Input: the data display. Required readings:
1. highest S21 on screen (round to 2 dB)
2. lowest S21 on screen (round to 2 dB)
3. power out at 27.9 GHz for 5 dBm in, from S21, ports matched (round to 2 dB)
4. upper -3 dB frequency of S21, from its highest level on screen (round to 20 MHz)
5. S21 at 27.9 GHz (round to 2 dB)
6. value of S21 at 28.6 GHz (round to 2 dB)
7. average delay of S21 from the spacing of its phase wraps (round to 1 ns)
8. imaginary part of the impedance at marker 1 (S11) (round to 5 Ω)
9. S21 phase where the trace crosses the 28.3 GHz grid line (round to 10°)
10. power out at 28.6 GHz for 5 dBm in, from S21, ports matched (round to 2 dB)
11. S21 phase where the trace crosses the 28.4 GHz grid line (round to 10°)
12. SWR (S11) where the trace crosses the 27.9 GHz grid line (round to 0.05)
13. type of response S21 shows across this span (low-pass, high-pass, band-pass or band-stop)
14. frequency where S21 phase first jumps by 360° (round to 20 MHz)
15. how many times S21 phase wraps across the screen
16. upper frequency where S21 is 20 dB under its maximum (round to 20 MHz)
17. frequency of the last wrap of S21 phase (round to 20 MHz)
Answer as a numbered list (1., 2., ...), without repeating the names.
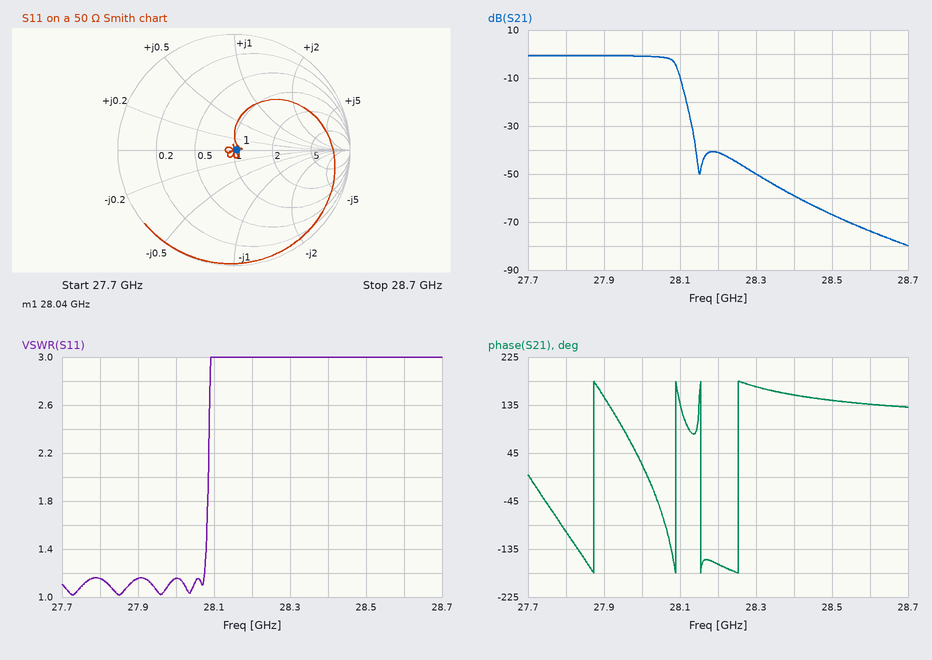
1. 0 dB
2. -80 dB
3. 4 dBm
4. 28.08 GHz
5. 0 dB
6. -74 dB
7. 8 ns
8. 0 Ω
9. 170°
10. -68 dBm
11. 150°
12. 1.15
13. low-pass
14. 27.88 GHz
15. 4
16. 28.12 GHz
17. 28.26 GHz
